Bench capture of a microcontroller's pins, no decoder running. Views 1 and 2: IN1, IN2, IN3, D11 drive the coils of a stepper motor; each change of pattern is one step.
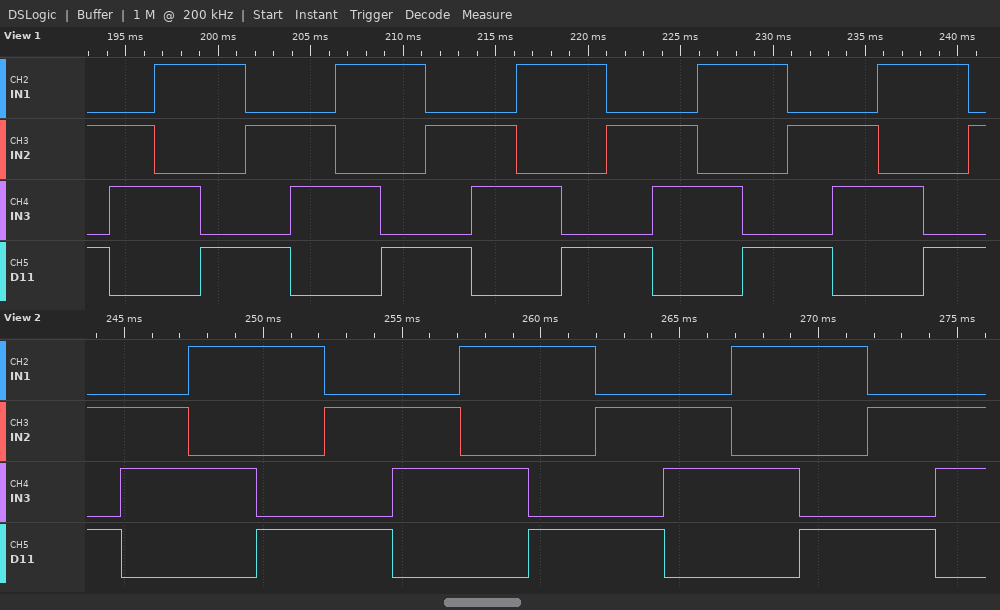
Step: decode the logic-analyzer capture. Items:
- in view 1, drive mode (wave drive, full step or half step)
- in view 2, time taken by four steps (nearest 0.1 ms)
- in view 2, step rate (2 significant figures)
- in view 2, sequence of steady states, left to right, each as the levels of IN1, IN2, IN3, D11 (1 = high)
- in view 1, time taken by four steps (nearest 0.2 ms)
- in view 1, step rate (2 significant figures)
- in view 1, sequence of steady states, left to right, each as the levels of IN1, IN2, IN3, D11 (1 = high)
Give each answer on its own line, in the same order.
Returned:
full step
9.8 ms
410 steps/s
0101 0110 1010 1001 0101 0110 1010 1001 0101 0110 1010 1001 0101 0110
9.8 ms
410 steps/s
0101 0110 1010 1001 0101 0110 1010 1001 0101 0110 1010 1001 0101 0110 1010 1001 0101 0110 1010 1001 0101
